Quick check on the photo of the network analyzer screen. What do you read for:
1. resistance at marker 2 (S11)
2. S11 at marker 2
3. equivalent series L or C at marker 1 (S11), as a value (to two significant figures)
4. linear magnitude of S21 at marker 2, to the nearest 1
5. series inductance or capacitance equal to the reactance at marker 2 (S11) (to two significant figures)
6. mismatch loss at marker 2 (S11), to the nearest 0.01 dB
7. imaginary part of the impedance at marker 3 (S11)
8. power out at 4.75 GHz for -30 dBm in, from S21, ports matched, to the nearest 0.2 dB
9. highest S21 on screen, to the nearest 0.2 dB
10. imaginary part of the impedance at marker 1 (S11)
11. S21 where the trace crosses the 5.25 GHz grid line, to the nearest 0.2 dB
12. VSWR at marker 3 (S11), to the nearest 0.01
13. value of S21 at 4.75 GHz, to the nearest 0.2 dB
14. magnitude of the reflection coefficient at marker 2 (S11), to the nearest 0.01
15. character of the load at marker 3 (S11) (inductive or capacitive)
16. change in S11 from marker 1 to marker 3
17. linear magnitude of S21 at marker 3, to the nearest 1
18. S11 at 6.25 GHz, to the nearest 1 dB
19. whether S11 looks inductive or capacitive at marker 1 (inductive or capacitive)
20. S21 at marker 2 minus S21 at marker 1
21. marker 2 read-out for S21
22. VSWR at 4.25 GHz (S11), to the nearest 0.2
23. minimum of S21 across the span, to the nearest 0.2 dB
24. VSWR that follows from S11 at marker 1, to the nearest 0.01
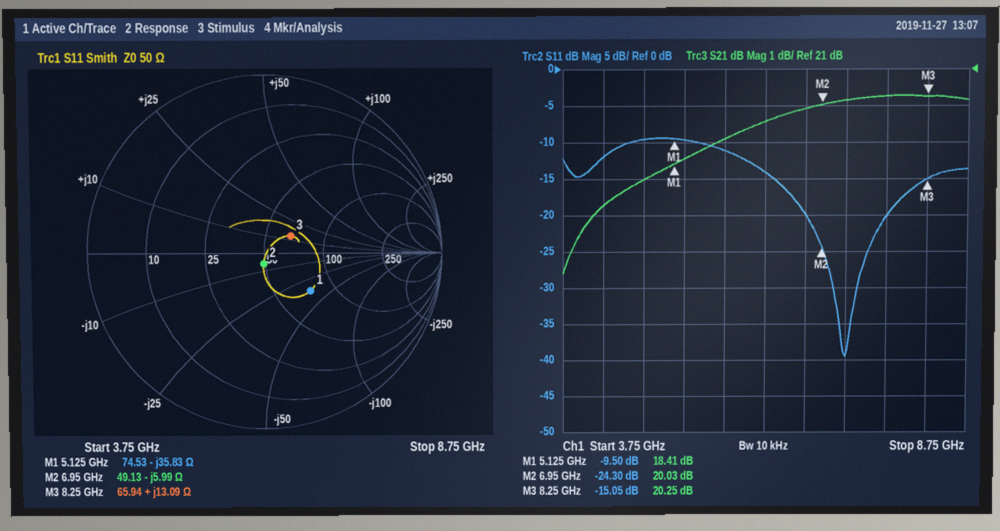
49.13 Ω
-24.30 dB
870 fF
10
3.8 pF
0.02 dB
+13.09 Ω
-12.0 dBm
20.2 dB
-35.83 Ω
18.6 dB
1.43
18.0 dB
0.06
inductive
-5.55 dB
10
-14 dB
capacitive
1.62 dB
20.03 dB
1.6
15.4 dB
2.01
